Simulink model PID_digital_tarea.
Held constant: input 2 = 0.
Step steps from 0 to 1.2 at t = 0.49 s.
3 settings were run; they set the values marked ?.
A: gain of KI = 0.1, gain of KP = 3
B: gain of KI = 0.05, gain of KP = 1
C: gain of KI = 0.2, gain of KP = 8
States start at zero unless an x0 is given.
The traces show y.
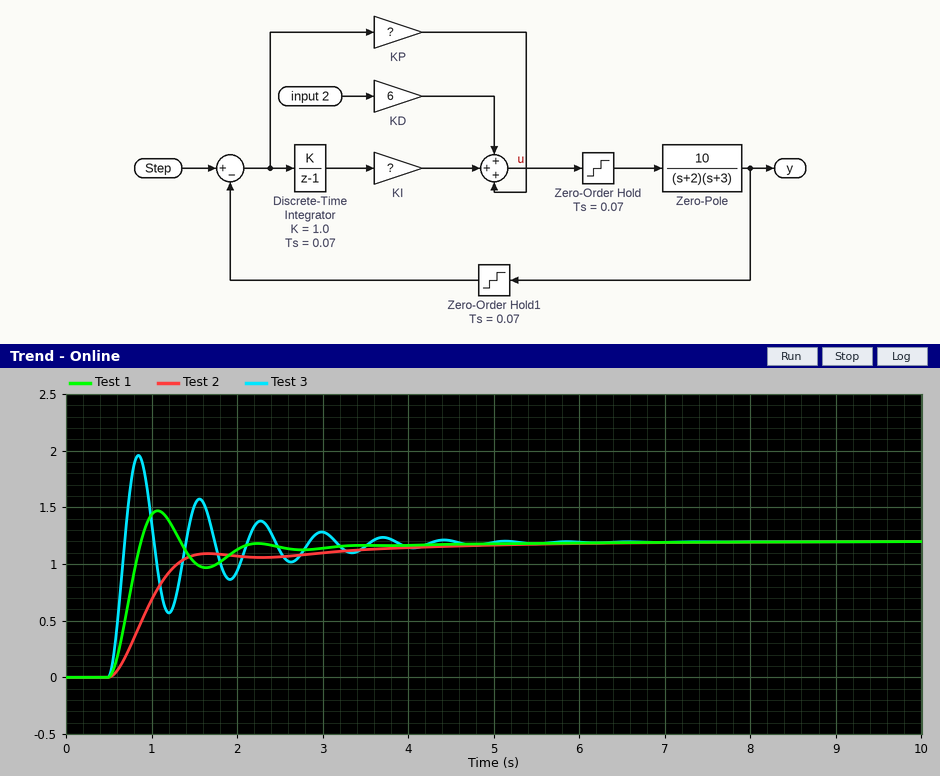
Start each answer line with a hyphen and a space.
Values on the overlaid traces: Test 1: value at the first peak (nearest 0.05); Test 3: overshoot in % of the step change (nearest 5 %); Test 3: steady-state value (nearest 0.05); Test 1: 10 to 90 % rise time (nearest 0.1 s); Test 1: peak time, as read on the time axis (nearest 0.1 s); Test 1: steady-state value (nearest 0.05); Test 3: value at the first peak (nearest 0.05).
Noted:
- 1.45
- 65 %
- 1.20
- 0.3 s
- 1.1 s
- 1.20
- 1.95
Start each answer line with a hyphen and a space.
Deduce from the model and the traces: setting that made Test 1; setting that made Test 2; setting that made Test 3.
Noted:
- A
- B
- C
